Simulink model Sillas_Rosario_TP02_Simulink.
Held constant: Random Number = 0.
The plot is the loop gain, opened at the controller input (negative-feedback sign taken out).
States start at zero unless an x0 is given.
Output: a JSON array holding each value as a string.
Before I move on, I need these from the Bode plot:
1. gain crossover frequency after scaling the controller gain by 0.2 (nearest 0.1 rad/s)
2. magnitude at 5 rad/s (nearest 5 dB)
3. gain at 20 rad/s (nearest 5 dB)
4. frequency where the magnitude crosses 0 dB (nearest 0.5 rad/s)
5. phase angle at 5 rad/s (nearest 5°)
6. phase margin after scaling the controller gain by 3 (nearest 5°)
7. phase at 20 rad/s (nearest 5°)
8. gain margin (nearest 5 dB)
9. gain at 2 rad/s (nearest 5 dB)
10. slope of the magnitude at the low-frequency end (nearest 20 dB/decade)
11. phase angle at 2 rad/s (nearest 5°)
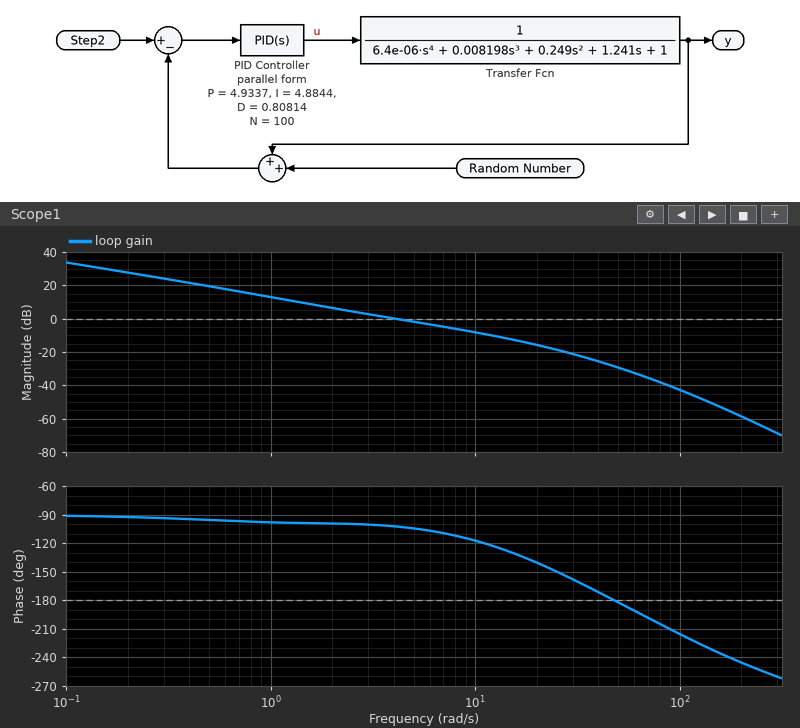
["0.9 rad/s", "0 dB", "-15 dB", "4.0 rad/s", "-105°", "60°", "-140°", "30 dB", "5 dB", "-20 dB/decade", "-100°"]
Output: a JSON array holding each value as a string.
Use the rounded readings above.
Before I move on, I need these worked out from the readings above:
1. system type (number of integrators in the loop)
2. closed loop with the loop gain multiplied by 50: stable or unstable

["1", "unstable"]
